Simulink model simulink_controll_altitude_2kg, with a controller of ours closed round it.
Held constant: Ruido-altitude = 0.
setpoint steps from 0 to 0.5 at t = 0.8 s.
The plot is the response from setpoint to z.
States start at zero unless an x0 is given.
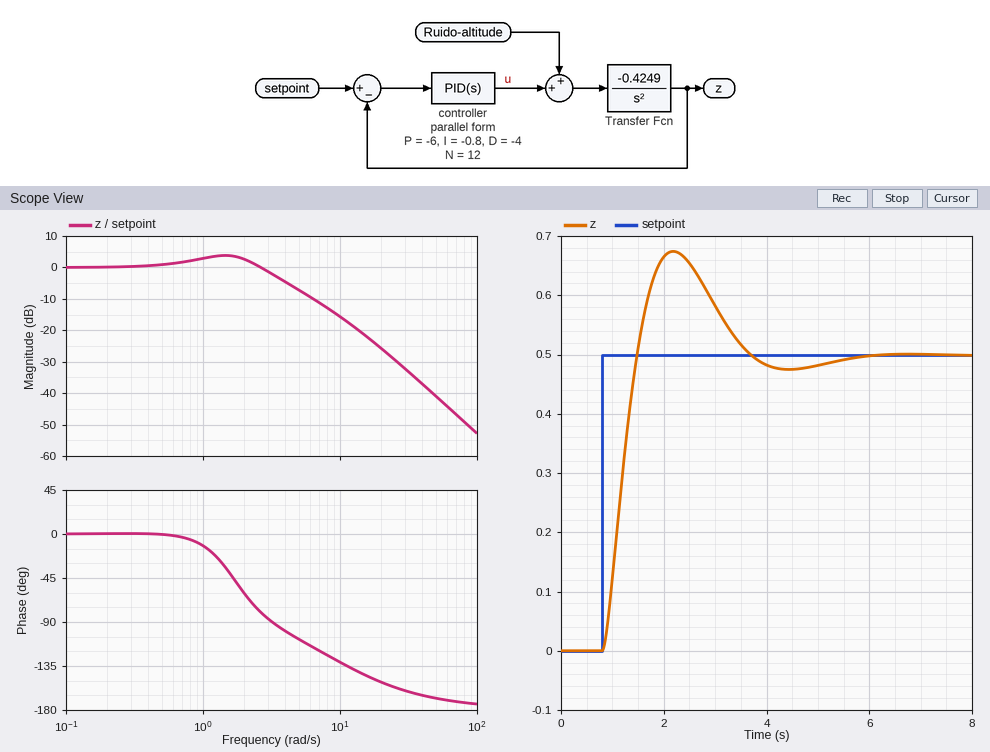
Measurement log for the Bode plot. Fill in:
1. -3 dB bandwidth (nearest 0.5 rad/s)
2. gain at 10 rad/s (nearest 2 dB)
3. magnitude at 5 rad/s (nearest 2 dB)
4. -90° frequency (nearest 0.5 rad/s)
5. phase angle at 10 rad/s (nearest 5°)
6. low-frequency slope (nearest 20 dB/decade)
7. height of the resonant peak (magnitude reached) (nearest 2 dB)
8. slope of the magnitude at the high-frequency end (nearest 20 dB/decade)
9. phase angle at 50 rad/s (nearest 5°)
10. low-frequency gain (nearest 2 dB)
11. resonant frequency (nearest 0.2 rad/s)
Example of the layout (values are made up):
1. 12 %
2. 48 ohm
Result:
1. 3.5 rad/s
2. -16 dB
3. -8 dB
4. 3.0 rad/s
5. -130°
6. 0 dB/decade
7. 4 dB
8. -40 dB/decade
9. -170°
10. 0 dB
11. 1.4 rad/s
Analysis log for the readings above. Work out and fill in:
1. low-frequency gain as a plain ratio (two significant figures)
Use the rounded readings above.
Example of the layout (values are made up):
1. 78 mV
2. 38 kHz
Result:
1. 1.0
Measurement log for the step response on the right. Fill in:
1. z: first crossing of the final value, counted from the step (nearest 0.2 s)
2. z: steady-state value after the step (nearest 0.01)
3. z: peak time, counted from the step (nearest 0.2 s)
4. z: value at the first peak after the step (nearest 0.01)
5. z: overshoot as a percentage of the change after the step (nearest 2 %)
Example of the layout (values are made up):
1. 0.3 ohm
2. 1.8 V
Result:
1. 0.6 s
2. 0.50
3. 1.4 s
4. 0.67
5. 34 %
